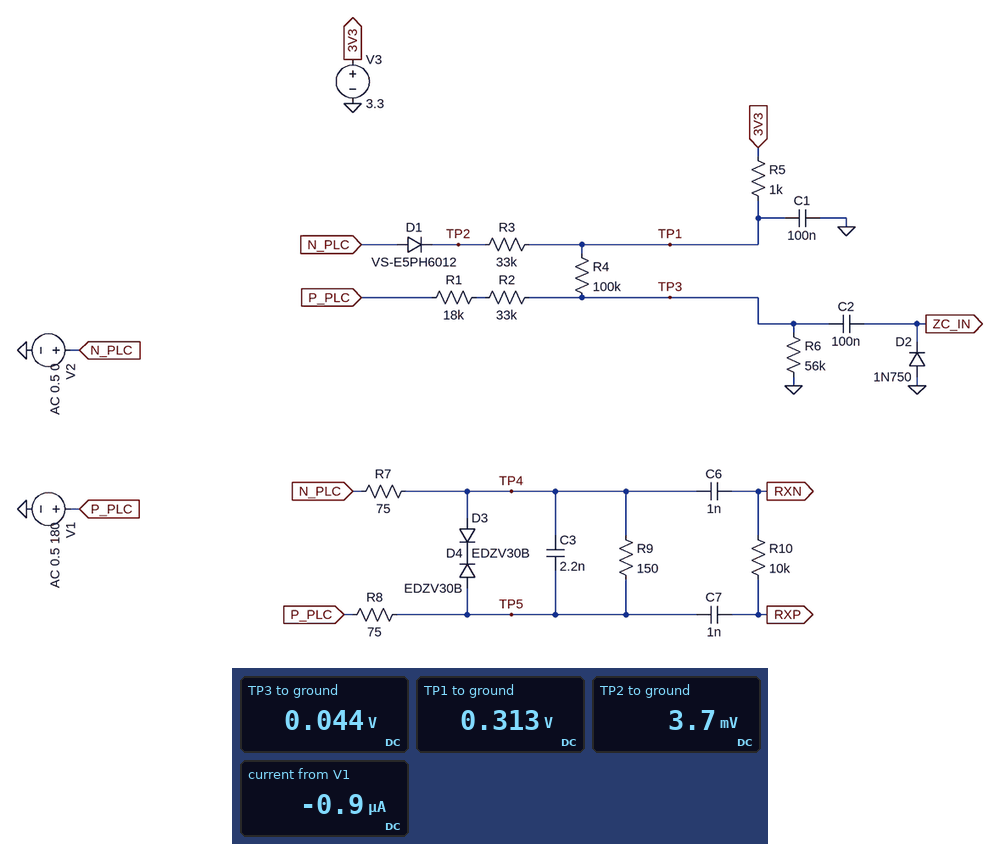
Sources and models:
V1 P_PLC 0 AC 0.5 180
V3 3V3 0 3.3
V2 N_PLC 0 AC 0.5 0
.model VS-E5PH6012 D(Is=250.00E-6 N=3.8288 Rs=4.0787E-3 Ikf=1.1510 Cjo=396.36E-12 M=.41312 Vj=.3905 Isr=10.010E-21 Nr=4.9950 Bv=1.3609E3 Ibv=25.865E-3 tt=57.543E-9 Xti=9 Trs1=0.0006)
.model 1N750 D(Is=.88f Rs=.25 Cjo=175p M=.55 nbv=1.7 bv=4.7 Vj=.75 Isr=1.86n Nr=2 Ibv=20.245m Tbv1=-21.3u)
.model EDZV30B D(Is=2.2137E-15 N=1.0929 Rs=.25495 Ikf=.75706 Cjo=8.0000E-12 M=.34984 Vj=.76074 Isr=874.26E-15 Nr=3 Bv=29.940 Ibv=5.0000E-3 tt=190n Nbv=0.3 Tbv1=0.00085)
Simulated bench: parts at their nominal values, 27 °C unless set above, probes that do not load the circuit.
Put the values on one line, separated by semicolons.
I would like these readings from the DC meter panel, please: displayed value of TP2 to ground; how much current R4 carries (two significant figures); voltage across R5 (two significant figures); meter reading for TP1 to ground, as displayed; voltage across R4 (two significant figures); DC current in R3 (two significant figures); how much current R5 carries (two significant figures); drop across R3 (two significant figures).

3.7 mV; 2.7 µA; 3.0 V; 0.313 V; 270 mV; 9.4 µA; 3.0 mA; 310 mV
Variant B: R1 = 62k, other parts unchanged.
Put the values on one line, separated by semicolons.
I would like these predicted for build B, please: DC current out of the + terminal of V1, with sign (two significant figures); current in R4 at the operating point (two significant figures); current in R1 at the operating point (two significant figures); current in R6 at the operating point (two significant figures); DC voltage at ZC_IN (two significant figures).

-520 nA; 2.6 µA; 520 nA; 890 nA; 50 mV
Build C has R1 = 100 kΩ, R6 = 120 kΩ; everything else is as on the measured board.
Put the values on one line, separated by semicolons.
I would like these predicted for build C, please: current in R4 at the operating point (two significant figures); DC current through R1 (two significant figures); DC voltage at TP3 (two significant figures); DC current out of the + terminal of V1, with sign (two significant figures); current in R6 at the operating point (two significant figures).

2.5 µA; 450 nA; 60 mV; -450 nA; 500 nA
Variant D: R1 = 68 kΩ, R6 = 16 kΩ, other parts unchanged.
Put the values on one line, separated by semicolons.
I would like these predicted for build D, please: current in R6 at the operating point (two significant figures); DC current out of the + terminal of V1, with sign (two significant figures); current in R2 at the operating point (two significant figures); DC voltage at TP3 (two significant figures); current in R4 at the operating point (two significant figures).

1.9 µA; -300 nA; 300 nA; 30 mV; 2.8 µA
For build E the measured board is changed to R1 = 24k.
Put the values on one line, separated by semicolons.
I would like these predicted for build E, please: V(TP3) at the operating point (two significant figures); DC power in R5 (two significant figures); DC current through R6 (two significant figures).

45 mV; 8.9 mW; 810 nA
